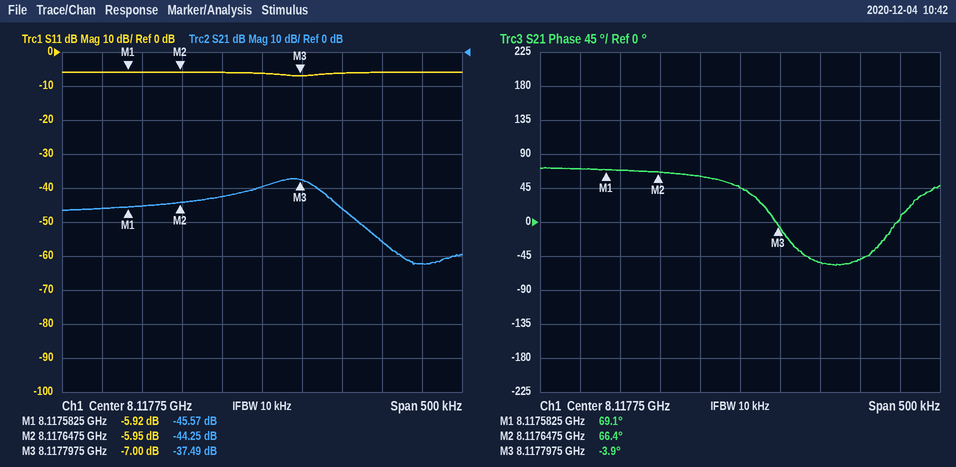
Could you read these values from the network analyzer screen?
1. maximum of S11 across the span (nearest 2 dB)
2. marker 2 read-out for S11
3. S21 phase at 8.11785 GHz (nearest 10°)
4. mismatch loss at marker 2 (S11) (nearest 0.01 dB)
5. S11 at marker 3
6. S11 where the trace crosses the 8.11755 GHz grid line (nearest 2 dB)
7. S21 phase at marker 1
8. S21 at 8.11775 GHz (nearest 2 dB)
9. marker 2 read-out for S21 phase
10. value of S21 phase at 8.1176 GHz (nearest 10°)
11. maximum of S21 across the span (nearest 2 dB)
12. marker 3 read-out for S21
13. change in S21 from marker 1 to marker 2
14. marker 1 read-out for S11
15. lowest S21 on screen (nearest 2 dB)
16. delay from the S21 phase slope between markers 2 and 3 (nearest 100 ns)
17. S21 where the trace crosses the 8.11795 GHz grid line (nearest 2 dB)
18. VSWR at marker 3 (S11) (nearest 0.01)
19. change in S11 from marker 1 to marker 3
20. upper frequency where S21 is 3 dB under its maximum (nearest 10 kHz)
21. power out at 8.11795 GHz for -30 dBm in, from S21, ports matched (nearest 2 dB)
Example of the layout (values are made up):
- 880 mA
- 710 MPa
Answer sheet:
- -6 dB
- -5.95 dB
- -50°
- 1.27 dB
- -7.00 dB
- -6 dB
- 69.1°
- -40 dB
- 66.4°
- 70°
- -38 dB
- -37.49 dB
- 1.32 dB
- -5.92 dB
- -62 dB
- 1.3 µs
- -62 dB
- 2.61
- -1.08 dB
- 8.11782 GHz
- -92 dBm
